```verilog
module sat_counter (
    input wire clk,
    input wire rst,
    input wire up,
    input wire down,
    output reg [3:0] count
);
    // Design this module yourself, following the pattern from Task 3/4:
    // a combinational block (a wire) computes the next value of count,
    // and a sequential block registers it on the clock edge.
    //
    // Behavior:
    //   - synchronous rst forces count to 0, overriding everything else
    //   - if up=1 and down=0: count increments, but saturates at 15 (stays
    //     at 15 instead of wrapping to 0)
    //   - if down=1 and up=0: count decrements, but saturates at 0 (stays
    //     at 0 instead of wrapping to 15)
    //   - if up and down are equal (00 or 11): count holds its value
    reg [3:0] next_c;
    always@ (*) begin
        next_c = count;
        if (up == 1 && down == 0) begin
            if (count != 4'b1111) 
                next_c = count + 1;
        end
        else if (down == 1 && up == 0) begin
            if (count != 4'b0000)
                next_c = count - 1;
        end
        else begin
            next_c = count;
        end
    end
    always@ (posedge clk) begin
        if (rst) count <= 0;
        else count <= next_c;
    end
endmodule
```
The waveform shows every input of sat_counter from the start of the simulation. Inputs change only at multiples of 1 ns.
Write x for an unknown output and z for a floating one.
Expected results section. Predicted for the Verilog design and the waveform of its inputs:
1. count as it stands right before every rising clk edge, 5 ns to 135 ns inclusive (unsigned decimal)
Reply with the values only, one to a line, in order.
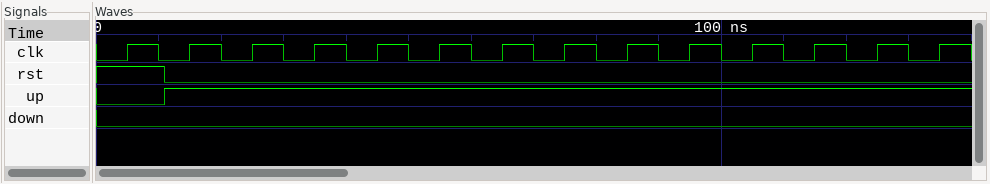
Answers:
x, 0, 1, 2, 3, 4, 5, 6, 7, 8, 9, 10, 11, 12
